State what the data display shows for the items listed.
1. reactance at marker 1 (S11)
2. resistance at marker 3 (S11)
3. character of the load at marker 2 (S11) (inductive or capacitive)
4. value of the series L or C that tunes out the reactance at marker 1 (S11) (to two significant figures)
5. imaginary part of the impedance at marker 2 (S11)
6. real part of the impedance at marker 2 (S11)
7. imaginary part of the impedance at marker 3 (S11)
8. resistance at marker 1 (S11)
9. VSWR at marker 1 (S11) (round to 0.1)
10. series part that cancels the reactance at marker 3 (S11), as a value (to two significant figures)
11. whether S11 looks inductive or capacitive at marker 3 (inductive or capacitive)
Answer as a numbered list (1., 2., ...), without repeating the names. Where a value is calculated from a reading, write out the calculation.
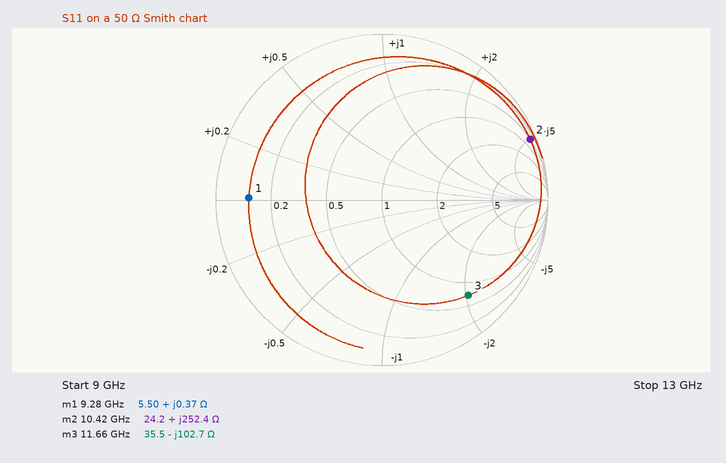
1. +0.37 Ω
2. 35.5 Ω
3. inductive
4. C = 1/(2π × 9.28 GHz × 0.37 Ω) ≈ 46 pF
5. +252.4 Ω
6. 24.2 Ω
7. -102.7 Ω
8. 5.50 Ω
9. 9.1
10. L = 102.7 Ω/(2π × 11.66 GHz) ≈ 1.4 nH
11. capacitive
